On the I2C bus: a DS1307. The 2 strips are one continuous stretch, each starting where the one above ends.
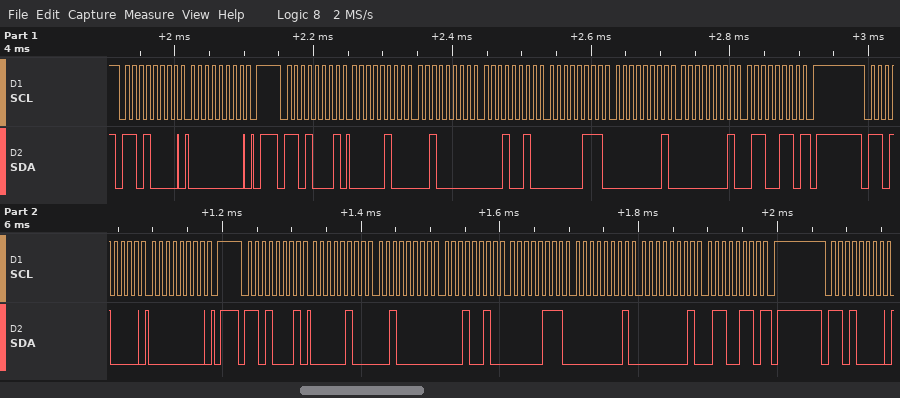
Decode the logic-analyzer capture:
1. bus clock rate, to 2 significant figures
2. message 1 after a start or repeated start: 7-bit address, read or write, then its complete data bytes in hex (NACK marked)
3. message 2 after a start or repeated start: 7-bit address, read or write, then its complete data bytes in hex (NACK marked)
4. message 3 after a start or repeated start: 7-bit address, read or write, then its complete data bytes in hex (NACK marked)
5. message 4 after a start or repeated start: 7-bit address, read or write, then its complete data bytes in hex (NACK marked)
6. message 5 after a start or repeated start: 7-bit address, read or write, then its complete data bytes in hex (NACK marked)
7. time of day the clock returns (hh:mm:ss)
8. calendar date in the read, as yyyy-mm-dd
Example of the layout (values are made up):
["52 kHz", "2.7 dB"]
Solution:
["100 kHz", "0x68 write: 00", "0x68 read: 04 20 12 07 01 01 66 NACK", "0x68 write: 00", "0x68 read: 04 20 12 07 01 01 66 NACK", "0x68 write", "12:20:04", "2066-01-01"]
